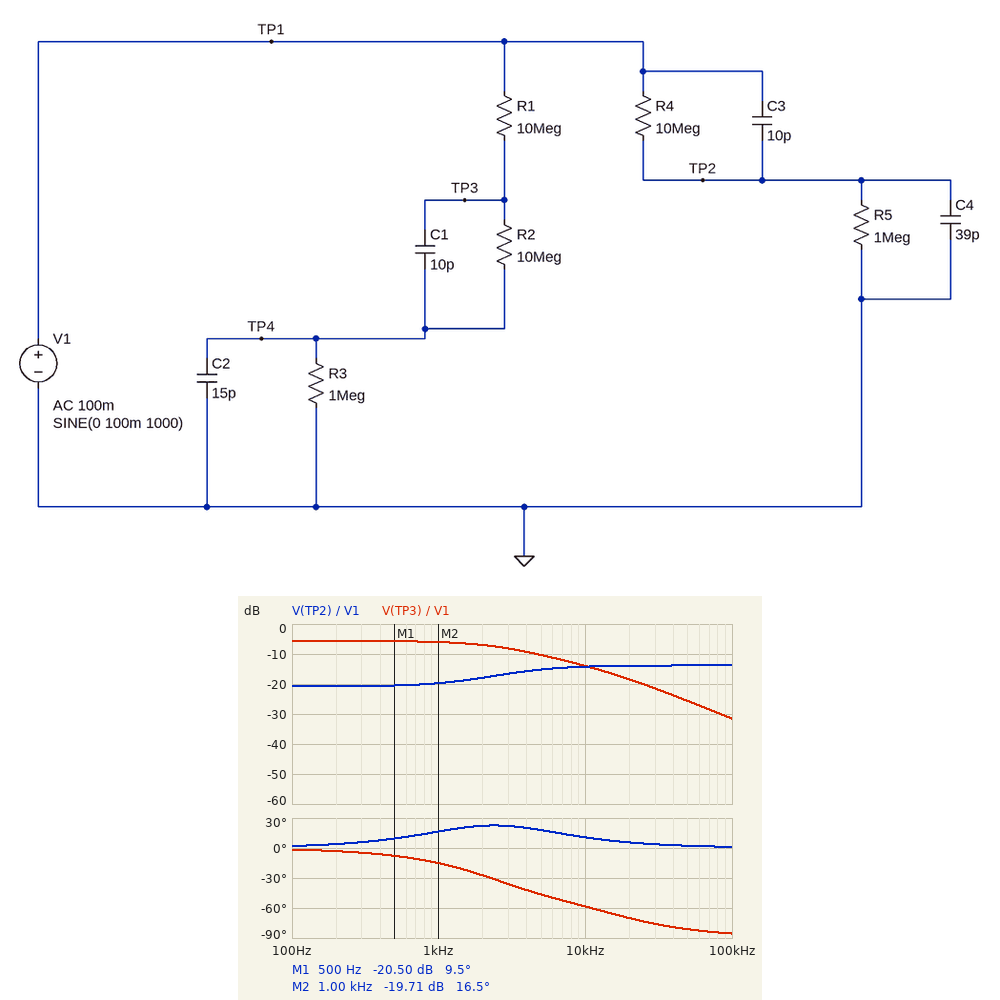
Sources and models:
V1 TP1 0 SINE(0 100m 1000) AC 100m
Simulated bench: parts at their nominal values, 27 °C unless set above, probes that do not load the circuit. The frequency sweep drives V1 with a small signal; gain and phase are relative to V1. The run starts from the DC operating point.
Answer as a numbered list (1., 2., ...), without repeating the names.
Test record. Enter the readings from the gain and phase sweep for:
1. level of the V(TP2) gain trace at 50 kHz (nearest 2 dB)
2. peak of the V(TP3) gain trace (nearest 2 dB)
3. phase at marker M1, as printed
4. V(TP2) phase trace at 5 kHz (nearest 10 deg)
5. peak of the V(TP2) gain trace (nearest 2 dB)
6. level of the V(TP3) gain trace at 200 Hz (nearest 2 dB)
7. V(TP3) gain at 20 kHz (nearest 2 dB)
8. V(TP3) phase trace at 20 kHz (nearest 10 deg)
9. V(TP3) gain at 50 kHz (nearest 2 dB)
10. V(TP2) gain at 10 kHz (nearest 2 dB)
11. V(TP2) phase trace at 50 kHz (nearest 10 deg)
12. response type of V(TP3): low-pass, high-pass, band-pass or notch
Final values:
1. -14 dB
2. -6 dB
3. 9.5 deg
4. 20 deg
5. -14 dB
6. -6 dB
7. -18 dB
8. -70 deg
9. -26 dB
10. -14 dB
11. 0 deg
12. low-pass
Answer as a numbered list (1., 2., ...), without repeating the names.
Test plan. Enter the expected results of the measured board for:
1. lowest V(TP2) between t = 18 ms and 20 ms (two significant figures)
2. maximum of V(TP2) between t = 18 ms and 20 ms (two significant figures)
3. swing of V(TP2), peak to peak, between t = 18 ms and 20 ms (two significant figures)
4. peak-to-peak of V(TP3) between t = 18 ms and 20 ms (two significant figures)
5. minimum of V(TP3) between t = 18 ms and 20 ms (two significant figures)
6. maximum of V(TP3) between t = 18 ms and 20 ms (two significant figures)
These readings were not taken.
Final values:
1. -10 mV
2. 10 mV
3. 21 mV
4. 100 mV
5. -50 mV
6. 50 mV
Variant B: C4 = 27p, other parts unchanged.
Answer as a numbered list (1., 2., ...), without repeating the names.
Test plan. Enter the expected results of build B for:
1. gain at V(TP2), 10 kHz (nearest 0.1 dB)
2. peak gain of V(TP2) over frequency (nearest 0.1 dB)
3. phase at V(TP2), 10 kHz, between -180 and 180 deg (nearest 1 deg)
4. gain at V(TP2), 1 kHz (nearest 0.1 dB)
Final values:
1. -12.1 dB
2. -11.4 dB
3. 16 deg
4. -19.6 dB
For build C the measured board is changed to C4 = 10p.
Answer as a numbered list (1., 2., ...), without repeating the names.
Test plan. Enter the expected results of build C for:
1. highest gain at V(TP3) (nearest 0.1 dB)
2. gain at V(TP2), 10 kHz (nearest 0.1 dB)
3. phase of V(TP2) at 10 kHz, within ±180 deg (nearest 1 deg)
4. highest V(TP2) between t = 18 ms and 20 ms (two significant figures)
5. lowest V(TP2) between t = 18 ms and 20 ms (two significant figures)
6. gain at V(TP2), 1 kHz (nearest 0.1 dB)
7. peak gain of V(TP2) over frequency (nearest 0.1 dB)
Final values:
1. -5.6 dB
2. -8.4 dB
3. 32 deg
4. 11 mV
5. -11 mV
6. -19.4 dB
7. -6.0 dB
